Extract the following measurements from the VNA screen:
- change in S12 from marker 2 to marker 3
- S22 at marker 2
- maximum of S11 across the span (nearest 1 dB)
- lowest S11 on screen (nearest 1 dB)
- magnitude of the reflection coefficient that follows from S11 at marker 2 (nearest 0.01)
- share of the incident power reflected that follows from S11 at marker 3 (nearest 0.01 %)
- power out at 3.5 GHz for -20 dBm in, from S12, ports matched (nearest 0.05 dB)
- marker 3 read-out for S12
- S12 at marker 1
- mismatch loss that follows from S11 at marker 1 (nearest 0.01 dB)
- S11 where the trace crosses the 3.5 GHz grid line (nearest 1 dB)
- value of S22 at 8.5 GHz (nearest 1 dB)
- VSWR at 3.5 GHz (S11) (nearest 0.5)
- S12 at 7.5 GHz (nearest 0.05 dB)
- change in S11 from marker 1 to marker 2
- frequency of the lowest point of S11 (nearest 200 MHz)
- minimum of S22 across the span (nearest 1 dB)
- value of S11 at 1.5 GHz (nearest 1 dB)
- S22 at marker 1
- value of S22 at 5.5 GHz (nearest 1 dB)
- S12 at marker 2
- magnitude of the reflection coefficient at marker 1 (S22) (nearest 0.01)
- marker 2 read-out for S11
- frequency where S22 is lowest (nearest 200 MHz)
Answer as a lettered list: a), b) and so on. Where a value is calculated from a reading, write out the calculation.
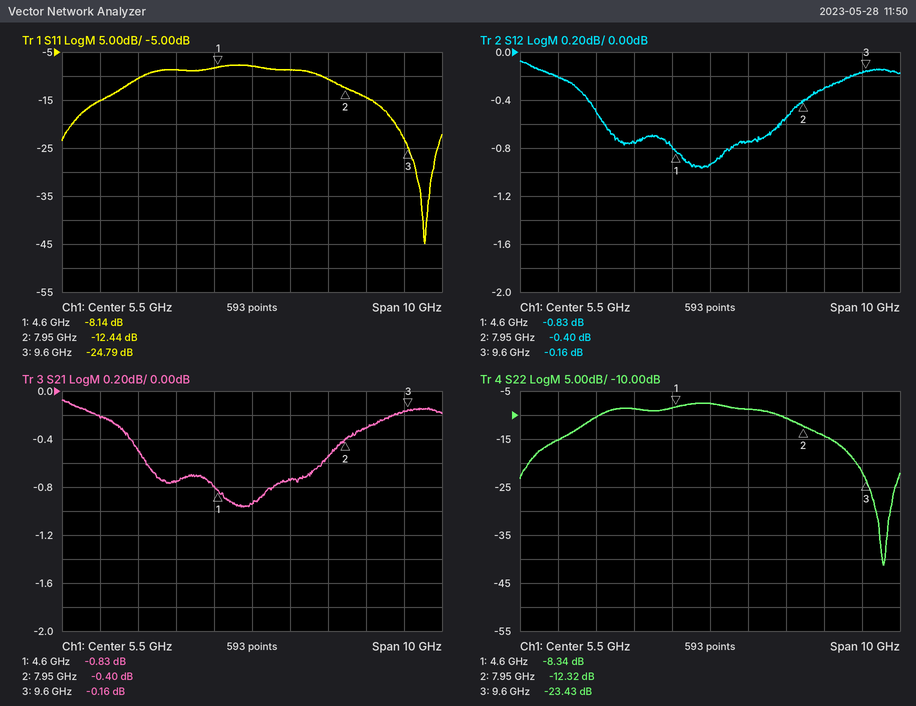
a) -0.16 − (-0.4) = 0.24 dB
b) -12.32 dB
c) -8 dB
d) -45 dB
e) 10^(-12.44/20) ≈ 0.24
f) 10^(-24.79/10) ≈ 0.33 %
g) -20 dBm + (-0.75 dB) = -20.75 dBm
h) -0.16 dB
i) -0.83 dB
j) −10 log10(1 − 10^(-8.14/10)) ≈ 0.72 dB
k) -9 dB
l) -14 dB
m) |Γ| = 10^(-9/20) = 0.3548; VSWR = (1 + 0.3548)/(1 − 0.3548) ≈ 2.10, so 2.0 to the nearest 0.5
n) -0.55 dB
o) -12.44 − (-8.14) = -4.30 dB
p) 10.0 GHz
q) -41 dB
r) -15 dB
s) -8.34 dB
t) -8 dB
u) -0.40 dB
v) 10^(-8.34/20) ≈ 0.38
w) -12.44 dB
x) 10.0 GHz
